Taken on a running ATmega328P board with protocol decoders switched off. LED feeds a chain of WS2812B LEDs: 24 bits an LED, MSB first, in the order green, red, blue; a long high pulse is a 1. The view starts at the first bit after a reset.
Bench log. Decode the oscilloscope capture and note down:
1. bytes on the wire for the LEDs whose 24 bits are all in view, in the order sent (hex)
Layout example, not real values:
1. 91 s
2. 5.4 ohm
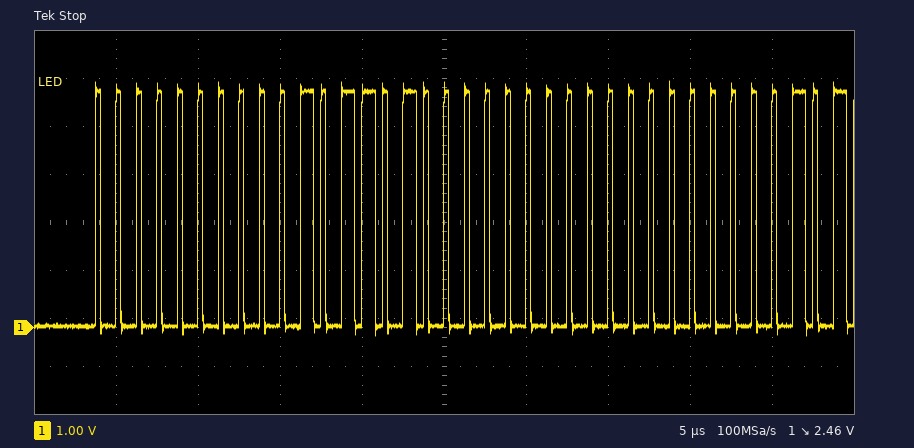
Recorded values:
1. 00 2D 00
